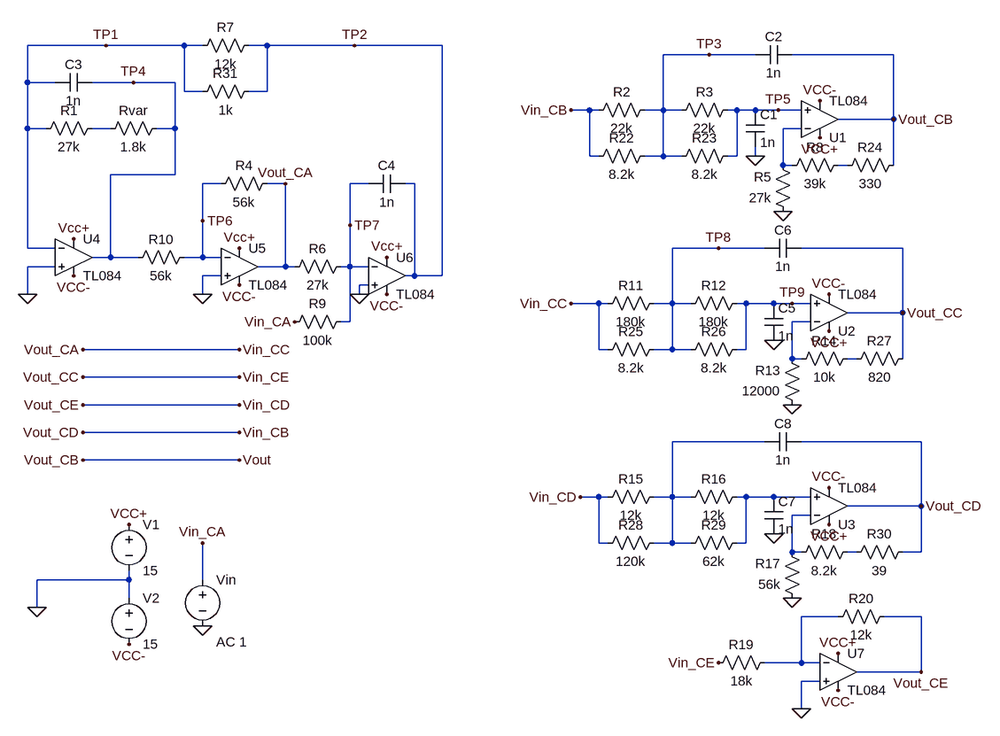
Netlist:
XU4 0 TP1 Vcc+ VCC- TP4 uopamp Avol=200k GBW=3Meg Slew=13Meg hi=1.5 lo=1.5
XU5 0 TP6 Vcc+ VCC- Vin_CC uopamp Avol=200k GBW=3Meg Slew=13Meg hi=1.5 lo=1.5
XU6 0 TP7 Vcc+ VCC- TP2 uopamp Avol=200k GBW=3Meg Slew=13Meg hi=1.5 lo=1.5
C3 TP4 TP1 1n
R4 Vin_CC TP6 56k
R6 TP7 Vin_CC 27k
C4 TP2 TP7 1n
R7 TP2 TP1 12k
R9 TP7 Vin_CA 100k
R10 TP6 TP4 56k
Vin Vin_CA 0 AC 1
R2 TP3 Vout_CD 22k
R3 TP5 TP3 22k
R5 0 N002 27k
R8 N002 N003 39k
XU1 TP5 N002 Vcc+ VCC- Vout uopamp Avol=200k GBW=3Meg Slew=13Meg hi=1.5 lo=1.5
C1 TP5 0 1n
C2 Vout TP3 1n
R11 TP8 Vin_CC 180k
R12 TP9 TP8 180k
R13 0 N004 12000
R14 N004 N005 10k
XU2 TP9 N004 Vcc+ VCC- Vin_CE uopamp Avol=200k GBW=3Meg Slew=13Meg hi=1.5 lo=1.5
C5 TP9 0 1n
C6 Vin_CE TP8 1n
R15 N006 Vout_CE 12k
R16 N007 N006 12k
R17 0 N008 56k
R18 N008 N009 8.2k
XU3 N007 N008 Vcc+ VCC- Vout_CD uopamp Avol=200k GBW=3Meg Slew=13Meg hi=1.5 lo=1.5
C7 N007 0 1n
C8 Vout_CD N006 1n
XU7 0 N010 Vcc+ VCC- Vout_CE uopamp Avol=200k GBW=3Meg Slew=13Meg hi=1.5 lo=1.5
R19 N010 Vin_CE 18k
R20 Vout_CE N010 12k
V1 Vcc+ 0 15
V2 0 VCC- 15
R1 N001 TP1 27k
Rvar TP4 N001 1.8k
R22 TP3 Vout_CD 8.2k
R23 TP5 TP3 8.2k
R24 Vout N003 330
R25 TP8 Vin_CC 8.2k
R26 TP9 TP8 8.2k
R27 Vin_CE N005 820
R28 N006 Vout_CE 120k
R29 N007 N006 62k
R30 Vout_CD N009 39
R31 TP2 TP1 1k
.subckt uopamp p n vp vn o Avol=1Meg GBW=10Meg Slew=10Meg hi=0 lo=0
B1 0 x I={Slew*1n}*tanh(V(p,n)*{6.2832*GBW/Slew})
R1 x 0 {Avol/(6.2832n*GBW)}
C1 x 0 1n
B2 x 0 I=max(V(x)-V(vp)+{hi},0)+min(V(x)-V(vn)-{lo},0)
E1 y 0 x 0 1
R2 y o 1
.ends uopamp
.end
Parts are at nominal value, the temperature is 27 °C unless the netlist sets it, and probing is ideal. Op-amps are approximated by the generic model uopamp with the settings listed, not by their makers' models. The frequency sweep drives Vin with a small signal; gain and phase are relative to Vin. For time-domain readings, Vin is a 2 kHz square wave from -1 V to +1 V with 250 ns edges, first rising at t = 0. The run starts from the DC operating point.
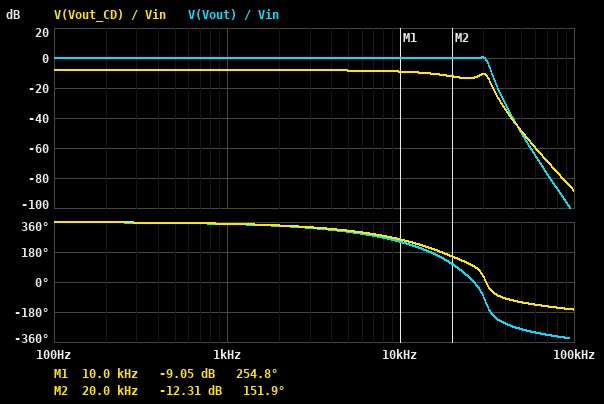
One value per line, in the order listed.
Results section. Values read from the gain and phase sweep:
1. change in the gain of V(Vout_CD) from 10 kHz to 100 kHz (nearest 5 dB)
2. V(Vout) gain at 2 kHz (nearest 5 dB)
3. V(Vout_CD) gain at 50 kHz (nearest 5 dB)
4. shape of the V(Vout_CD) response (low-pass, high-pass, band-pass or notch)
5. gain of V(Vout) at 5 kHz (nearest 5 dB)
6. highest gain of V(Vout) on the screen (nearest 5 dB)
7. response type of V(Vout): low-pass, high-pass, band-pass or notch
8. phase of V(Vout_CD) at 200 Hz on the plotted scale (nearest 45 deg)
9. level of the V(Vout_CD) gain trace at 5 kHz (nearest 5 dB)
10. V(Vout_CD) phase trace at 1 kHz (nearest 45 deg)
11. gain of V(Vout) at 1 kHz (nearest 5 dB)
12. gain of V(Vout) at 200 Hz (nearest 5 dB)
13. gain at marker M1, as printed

-80 dB
0 dB
-50 dB
low-pass
0 dB
0 dB
low-pass
360 deg
-10 dB
360 deg
0 dB
0 dB
-9.05 dB
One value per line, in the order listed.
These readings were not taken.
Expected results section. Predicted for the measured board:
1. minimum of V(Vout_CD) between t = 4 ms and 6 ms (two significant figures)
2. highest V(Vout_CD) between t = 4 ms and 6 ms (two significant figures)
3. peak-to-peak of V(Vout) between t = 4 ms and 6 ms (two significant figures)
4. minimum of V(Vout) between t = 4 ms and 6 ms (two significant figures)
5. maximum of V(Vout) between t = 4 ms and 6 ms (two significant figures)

-430 mV
430 mV
2.8 V
-1.4 V
1.4 V
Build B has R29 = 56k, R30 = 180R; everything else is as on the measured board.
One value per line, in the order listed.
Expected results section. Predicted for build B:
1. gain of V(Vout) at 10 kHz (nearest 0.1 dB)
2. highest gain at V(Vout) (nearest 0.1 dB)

0 dB
0.6 dB
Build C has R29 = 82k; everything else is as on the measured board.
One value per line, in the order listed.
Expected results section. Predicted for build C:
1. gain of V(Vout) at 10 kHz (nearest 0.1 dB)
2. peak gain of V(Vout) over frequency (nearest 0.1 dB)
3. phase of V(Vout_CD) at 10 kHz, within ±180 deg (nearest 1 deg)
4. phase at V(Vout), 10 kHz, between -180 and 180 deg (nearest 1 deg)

-0.2 dB
0.1 dB
-106 deg
-120 deg
